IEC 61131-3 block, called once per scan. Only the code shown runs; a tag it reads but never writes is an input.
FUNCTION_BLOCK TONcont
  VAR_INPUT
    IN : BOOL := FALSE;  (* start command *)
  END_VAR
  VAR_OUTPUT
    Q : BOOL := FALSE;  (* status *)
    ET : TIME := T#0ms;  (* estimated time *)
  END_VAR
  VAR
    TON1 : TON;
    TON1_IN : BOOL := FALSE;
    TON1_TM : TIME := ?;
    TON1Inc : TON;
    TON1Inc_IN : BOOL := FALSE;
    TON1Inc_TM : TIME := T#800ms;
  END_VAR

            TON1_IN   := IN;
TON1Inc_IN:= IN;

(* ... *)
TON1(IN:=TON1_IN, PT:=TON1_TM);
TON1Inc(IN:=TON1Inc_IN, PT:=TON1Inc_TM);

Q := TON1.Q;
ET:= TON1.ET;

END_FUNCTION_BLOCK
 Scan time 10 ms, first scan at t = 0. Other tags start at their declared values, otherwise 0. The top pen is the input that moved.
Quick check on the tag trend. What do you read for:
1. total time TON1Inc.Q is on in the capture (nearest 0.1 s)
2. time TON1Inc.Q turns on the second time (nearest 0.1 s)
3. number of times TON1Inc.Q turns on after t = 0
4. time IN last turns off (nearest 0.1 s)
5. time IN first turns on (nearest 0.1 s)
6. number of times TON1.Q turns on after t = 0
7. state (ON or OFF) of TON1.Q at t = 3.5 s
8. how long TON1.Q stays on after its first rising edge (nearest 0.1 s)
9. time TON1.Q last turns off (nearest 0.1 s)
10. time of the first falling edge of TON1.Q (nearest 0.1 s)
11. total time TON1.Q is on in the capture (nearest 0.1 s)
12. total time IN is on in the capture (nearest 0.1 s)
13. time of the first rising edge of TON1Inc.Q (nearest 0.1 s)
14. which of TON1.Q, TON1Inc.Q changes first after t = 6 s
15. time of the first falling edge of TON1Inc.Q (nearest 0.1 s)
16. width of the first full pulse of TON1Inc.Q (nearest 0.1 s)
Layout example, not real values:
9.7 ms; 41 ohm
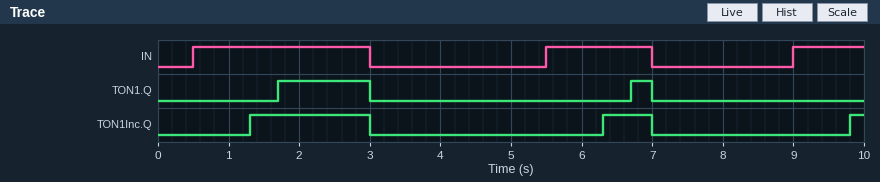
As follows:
2.6 s; 6.3 s; 3; 7.0 s; 0.5 s; 2; OFF; 1.3 s; 7.0 s; 3.0 s; 1.6 s; 5.0 s; 1.3 s; TON1Inc.Q; 3.0 s; 1.7 s
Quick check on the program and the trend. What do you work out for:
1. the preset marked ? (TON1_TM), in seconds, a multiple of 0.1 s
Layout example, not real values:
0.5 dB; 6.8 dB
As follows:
1.2 s
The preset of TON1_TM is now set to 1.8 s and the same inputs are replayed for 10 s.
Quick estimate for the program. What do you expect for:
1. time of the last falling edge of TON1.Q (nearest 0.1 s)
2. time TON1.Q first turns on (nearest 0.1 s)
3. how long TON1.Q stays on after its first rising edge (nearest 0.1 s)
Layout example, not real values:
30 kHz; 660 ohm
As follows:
3.0 s; 2.3 s; 0.7 s
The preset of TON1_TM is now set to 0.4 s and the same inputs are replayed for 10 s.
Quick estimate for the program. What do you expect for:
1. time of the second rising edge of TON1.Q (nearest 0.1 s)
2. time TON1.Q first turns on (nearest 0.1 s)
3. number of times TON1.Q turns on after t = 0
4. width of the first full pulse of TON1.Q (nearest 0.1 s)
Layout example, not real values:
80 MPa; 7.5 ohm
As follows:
5.9 s; 0.9 s; 3; 2.1 s
